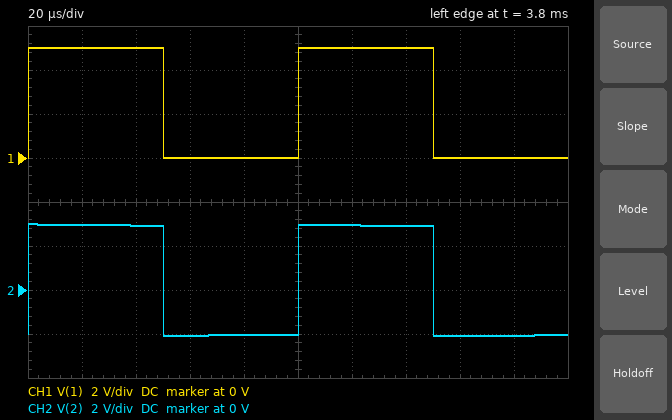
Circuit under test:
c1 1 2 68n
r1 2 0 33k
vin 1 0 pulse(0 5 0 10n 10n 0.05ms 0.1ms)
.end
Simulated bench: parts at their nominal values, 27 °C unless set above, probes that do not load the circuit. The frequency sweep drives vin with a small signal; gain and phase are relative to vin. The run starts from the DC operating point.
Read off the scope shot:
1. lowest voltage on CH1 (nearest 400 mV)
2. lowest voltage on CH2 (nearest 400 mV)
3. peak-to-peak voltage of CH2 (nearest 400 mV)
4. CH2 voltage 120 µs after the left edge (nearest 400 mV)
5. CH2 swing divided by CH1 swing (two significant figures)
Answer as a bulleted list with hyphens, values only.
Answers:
- 0 V
- -2.0 V
- 5.2 V
- 2.8 V
- 1.0
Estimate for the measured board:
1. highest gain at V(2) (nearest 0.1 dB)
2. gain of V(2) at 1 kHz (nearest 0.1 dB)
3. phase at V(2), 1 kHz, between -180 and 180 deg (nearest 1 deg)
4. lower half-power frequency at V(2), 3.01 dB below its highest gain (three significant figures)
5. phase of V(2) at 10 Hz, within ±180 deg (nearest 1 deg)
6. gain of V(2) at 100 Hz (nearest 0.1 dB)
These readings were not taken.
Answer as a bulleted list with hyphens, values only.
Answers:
- 0 dB
- 0 dB
- 4 deg
- 70.9 Hz
- 82 deg
- -1.8 dB
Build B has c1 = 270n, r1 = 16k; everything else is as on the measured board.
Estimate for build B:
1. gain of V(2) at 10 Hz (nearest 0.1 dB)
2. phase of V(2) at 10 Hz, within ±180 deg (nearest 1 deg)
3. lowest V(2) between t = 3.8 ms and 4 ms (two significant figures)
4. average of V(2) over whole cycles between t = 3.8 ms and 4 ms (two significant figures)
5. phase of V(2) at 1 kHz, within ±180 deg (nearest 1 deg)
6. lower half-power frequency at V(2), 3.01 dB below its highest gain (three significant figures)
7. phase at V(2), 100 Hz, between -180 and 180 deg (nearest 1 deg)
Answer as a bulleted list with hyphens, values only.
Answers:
- -11.6 dB
- 75 deg
- -1.5 V
- 1.0 V
- 2 deg
- 36.8 Hz
- 20 deg
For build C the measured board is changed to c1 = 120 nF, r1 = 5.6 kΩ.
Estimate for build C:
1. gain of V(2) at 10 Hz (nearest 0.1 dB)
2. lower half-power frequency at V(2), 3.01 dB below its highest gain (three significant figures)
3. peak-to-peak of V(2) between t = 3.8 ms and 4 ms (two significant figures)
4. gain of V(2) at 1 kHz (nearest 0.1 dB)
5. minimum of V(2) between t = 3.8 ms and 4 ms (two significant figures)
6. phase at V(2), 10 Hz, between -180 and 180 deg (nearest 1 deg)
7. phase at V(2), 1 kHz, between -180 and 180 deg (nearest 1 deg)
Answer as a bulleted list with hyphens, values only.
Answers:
- -27.5 dB
- 237 Hz
- 5.2 V
- -0.2 dB
- -2.6 V
- 88 deg
- 13 deg
